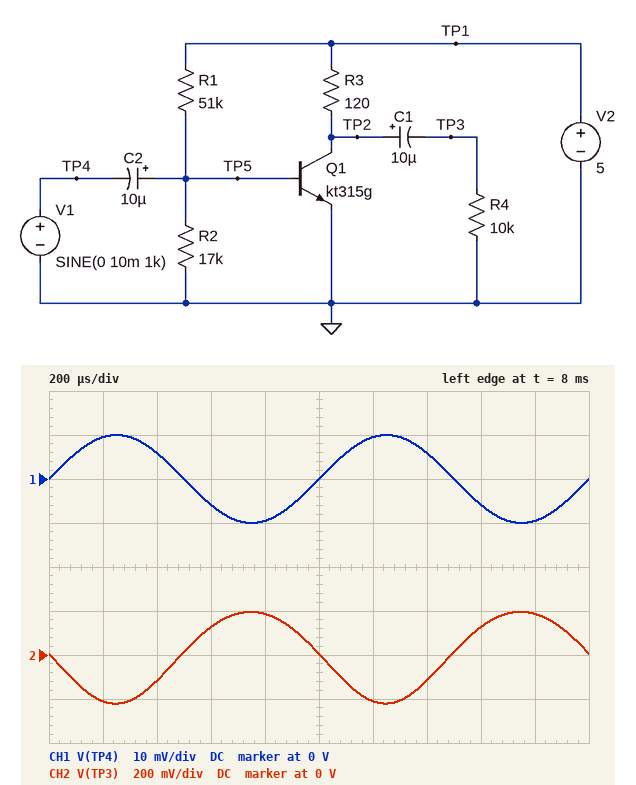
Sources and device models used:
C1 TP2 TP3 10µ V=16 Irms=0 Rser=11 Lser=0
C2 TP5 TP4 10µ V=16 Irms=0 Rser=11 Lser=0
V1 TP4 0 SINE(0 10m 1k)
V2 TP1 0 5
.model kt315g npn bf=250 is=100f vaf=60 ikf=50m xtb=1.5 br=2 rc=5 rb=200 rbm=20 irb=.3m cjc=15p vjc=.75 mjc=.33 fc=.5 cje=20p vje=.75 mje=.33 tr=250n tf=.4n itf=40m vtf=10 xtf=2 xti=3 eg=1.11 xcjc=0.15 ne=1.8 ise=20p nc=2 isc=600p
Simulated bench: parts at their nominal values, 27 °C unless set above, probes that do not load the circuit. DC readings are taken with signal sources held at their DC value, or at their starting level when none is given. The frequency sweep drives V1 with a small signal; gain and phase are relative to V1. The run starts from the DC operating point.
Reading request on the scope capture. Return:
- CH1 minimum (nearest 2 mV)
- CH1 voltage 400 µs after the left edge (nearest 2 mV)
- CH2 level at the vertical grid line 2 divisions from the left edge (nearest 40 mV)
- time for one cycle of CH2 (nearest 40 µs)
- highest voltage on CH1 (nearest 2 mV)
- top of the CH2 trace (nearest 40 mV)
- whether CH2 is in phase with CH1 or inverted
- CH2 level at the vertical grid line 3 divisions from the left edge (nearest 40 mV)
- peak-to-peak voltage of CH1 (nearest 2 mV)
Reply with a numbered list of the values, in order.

1. -10 mV
2. 6 mV
3. -120 mV
4. 1.00 ms
5. 10 mV
6. 200 mV
7. inverted
8. 120 mV
9. 20 mV
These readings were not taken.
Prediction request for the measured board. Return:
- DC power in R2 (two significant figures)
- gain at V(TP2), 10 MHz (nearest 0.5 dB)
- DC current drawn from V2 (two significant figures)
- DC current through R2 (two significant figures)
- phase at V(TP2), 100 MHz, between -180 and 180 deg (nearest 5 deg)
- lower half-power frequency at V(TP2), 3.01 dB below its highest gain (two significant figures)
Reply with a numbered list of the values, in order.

1. 25 µW
2. 21.0 dB
3. 6.3 mA
4. 38 µA
5. 65 deg
6. 20 Hz
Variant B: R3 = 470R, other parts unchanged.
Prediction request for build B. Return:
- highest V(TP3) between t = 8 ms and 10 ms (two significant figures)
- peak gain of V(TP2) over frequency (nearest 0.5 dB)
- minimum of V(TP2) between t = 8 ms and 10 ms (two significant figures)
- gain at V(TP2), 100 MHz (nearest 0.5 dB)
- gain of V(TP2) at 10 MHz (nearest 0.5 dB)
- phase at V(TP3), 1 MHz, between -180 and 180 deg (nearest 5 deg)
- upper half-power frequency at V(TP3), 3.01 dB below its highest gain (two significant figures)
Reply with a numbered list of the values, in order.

1. 700 mV
2. 37.0 dB
3. 1.4 V
4. 7.0 dB
5. 27.5 dB
6. 165 deg
7. 3.4 MHz
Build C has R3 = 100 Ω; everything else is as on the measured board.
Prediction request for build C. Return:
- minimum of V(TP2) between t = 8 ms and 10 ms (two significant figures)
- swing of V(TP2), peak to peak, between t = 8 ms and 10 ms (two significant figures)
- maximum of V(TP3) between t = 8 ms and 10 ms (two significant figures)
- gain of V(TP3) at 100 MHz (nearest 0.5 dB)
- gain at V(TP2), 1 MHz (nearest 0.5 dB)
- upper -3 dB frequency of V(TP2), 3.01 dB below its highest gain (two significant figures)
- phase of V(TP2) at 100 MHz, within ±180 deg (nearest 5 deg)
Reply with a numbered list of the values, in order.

1. 4.2 V
2. 350 mV
3. 160 mV
4. 2.5 dB
5. 24.5 dB
6. 6.9 MHz
7. 70 deg
